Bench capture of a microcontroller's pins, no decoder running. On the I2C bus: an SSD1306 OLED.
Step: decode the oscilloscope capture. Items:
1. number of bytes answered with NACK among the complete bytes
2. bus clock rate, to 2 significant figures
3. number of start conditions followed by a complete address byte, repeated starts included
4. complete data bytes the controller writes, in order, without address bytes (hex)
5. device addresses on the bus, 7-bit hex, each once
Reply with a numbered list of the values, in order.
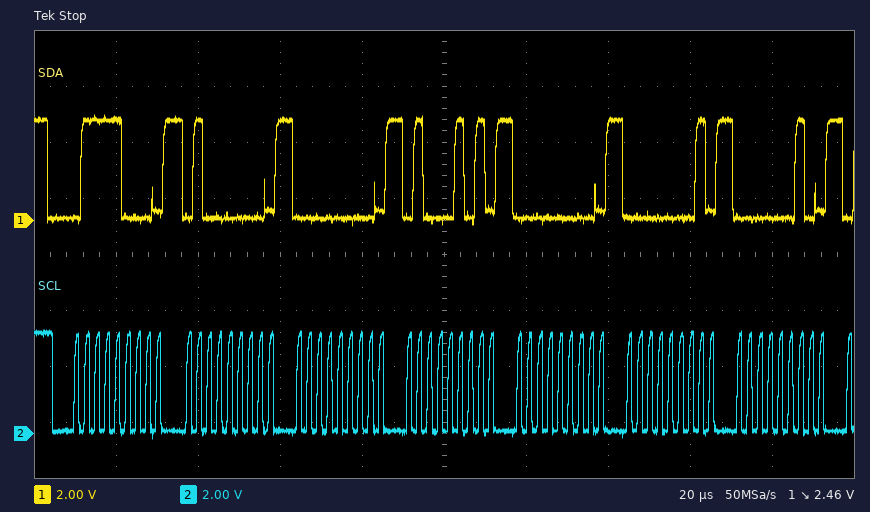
1. 0
2. 400 kHz
3. 1
4. 40 00 45 00 01 02
5. 0x3C
